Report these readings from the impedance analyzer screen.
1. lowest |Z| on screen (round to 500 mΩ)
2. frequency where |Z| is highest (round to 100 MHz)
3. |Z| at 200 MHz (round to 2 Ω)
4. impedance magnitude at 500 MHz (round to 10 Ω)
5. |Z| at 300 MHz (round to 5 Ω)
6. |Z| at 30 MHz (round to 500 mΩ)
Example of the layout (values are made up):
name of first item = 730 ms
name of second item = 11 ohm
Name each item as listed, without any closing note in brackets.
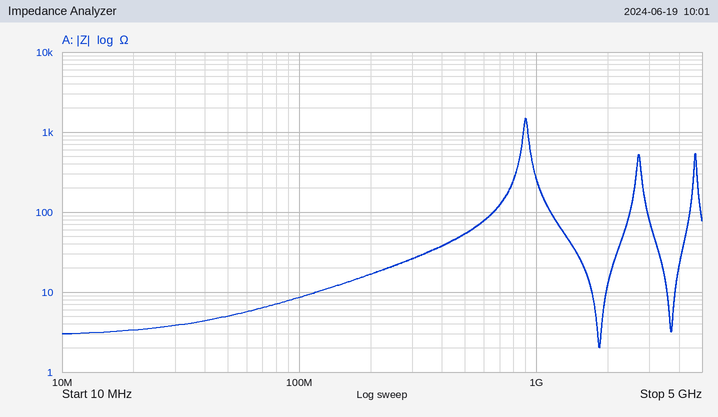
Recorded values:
lowest |Z| on screen = 2.0 Ω
frequency where |Z| is highest = 900 MHz
|Z| at 200 MHz = 16 Ω
impedance magnitude at 500 MHz = 50 Ω
|Z| at 300 MHz = 25 Ω
|Z| at 30 MHz = 4.0 Ω
